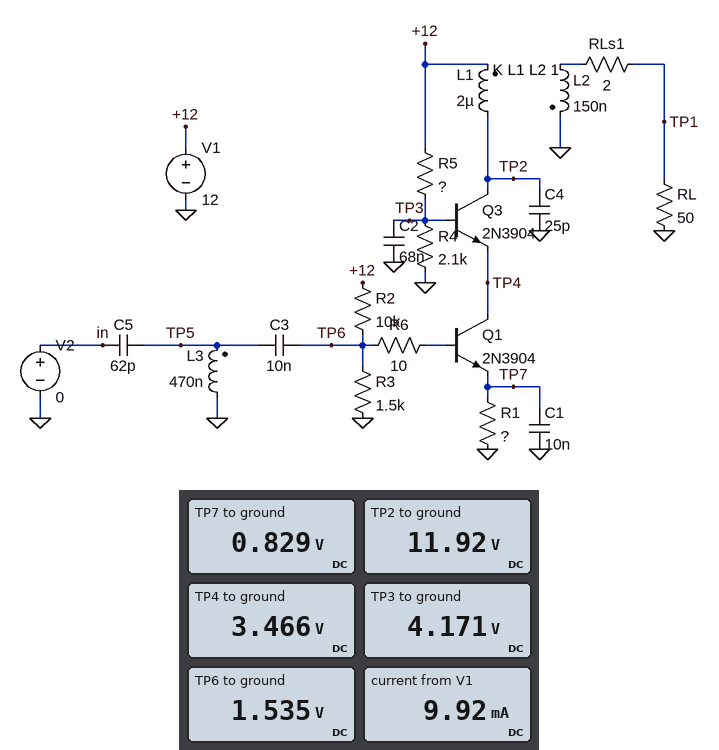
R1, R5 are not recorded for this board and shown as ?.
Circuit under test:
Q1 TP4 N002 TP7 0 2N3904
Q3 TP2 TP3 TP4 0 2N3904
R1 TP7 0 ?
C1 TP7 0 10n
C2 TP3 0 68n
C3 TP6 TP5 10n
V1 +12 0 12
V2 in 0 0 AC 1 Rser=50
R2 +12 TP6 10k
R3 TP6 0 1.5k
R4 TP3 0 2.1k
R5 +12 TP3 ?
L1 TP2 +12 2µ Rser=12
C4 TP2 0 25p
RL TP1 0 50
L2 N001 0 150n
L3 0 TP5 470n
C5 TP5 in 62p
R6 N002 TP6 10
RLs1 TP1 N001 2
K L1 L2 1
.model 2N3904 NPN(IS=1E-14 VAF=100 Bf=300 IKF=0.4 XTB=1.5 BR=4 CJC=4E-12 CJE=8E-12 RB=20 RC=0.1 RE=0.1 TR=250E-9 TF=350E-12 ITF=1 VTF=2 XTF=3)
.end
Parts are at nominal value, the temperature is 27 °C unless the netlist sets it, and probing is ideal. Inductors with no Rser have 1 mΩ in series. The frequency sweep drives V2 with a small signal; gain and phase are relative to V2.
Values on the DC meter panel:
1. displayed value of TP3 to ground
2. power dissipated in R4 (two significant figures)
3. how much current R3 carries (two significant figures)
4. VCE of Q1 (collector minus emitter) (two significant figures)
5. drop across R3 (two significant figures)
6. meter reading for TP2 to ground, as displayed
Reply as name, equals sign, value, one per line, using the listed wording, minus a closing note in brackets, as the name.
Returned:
displayed value of TP3 to ground = 4.171 V
power dissipated in R4 = 8.3 mW
how much current R3 carries = 1.0 mA
VCE of Q1 (collector minus emitter) = 2.6 V
drop across R3 = 1.5 V
meter reading for TP2 to ground, as displayed = 11.92 V
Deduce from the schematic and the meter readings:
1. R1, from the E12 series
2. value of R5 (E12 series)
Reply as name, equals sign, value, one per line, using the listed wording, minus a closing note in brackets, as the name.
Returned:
R1, from the E12 series = 120 Ω
value of R5 = 3.9 kΩ
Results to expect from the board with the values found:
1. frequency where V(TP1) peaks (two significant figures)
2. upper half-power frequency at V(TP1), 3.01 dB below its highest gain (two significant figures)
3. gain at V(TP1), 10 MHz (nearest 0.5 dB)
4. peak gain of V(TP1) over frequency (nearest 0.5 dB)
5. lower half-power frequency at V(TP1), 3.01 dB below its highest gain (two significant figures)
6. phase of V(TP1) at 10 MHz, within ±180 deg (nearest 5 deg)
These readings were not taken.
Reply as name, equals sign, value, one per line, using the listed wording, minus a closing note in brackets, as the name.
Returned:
frequency where V(TP1) peaks = 19 MHz
upper half-power frequency at V(TP1), 3.01 dB below its highest gain = 23 MHz
gain at V(TP1), 10 MHz = 4.0 dB
peak gain of V(TP1) over frequency = 32.5 dB
lower half-power frequency at V(TP1), 3.01 dB below its highest gain = 17 MHz
phase of V(TP1) at 10 MHz, within ±180 deg = 70 deg
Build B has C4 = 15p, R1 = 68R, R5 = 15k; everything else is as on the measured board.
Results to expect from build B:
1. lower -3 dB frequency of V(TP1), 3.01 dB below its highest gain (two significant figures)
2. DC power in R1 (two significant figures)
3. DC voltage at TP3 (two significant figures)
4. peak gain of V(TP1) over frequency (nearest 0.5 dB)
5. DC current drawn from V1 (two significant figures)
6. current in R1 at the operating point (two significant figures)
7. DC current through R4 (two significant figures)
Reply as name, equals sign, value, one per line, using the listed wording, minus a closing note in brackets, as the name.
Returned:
lower -3 dB frequency of V(TP1), 3.01 dB below its highest gain = 20 MHz
DC power in R1 = 5.9 mW
DC voltage at TP3 = 1.4 V
peak gain of V(TP1) over frequency = -5.5 dB
DC current drawn from V1 = 11 mA
current in R1 at the operating point = 9.3 mA
DC current through R4 = 680 µA
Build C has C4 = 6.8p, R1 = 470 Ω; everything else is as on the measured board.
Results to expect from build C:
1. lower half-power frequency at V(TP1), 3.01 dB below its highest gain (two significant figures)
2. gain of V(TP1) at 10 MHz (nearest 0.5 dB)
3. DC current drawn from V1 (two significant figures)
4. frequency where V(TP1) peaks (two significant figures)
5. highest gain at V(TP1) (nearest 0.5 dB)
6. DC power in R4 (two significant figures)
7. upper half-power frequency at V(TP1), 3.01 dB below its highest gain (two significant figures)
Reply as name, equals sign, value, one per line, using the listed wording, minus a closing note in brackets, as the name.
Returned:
lower half-power frequency at V(TP1), 3.01 dB below its highest gain = 21 MHz
gain of V(TP1) at 10 MHz = -9.5 dB
DC current drawn from V1 = 4.9 mA
frequency where V(TP1) peaks = 26 MHz
highest gain at V(TP1) = 21.5 dB
DC power in R4 = 8.4 mW
upper half-power frequency at V(TP1), 3.01 dB below its highest gain = 42 MHz
